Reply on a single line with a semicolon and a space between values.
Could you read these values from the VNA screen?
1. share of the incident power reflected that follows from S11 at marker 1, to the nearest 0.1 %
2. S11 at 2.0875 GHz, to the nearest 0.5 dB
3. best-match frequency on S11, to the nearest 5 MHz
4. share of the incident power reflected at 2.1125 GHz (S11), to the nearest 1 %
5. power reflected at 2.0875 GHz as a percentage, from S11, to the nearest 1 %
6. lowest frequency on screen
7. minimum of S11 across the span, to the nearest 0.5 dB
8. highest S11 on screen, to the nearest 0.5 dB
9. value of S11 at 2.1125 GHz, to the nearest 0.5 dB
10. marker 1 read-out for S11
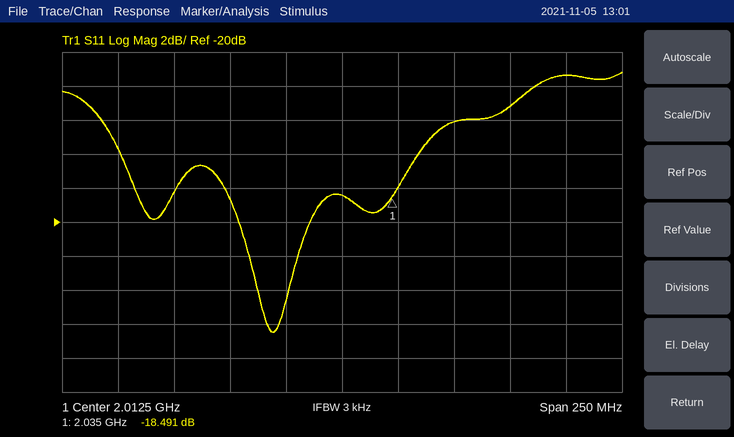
1.4 %; -13.0 dB; 1.980 GHz; 7 %; 5 %; 1.8875 GHz; -26.5 dB; -11.0 dB; -11.5 dB; -18.491 dB
